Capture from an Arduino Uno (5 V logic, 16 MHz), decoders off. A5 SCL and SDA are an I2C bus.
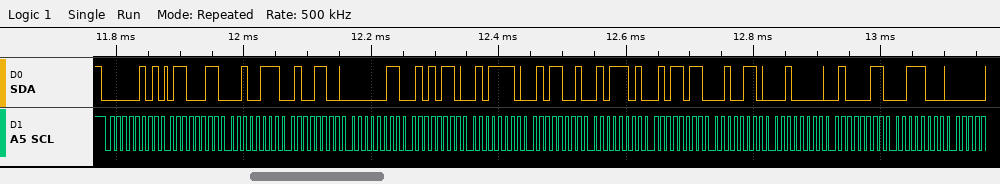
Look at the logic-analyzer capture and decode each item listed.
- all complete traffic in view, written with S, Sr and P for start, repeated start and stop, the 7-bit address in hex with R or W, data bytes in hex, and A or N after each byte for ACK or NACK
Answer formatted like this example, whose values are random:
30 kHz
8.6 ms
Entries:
S 02R A 63 A 27 A 4C A 03 A 56 A 5E A 59 A 5D A 5B A 26 A 20 A 43 A 38 A
